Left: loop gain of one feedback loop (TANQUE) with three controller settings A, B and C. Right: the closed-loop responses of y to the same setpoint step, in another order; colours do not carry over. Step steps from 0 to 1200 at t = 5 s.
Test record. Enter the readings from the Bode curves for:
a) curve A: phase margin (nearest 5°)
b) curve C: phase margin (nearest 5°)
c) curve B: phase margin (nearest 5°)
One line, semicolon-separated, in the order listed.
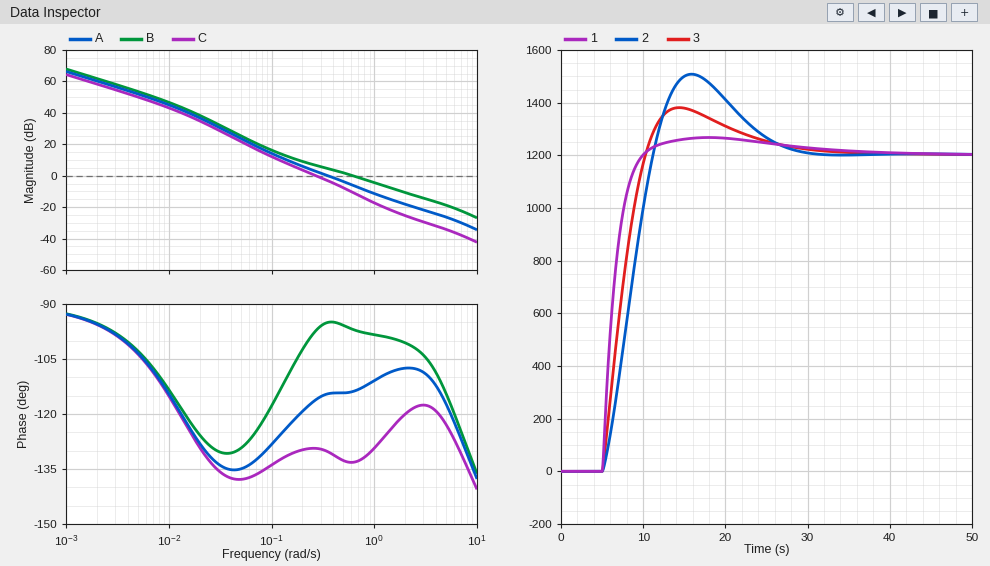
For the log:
65°; 50°; 85°
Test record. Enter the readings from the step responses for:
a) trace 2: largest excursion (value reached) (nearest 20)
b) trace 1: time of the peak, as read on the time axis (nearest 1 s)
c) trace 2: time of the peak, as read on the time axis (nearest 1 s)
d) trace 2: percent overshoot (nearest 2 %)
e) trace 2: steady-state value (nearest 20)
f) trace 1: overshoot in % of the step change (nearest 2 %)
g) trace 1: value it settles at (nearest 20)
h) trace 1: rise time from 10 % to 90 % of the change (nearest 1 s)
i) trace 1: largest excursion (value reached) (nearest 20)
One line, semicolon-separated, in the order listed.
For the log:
1500; 18 s; 16 s; 26 %; 1200; 6 %; 1200; 3 s; 1260
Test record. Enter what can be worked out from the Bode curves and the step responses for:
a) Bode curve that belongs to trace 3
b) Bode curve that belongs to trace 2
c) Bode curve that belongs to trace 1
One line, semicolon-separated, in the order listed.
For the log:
A; C; B
